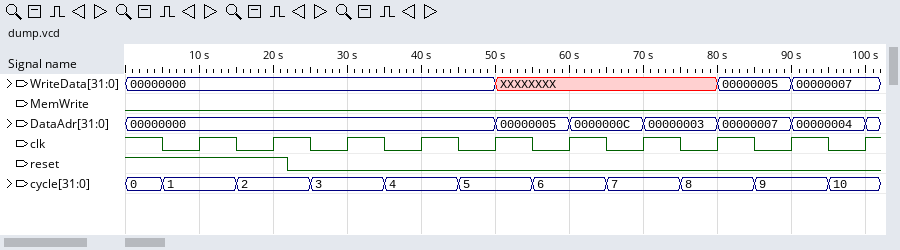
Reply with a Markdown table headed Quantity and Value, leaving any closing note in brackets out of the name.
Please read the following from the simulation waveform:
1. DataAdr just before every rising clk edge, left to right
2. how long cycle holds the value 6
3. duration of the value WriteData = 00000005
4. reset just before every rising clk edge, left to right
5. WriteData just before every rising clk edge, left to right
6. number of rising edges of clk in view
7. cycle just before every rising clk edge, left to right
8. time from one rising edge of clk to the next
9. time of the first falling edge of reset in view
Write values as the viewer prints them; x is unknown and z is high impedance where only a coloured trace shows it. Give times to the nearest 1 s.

| Quantity | Value |
|---|---|
| DataAdr just before every rising clk edge, left to right | 00000000, 00000000, 00000000, 00000000, 00000000, 00000005, 0000000C, 00000003, 00000007, 00000004 |
| how long cycle holds the value 6 | 10 s |
| duration of the value WriteData = 00000005 | 10 s |
| reset just before every rising clk edge, left to right | 1 1 0 0 0 0 0 0 0 0 |
| WriteData just before every rising clk edge, left to right | 00000000, 00000000, 00000000, 00000000, 00000000, XXXXXXXX, XXXXXXXX, XXXXXXXX, 00000005, 00000007 |
| number of rising edges of clk in view | 10 |
| cycle just before every rising clk edge, left to right | 1, 2, 3, 4, 5, 6, 7, 8, 9, 10 |
| time from one rising edge of clk to the next | 10 s |
| time of the first falling edge of reset in view | 22 s |
